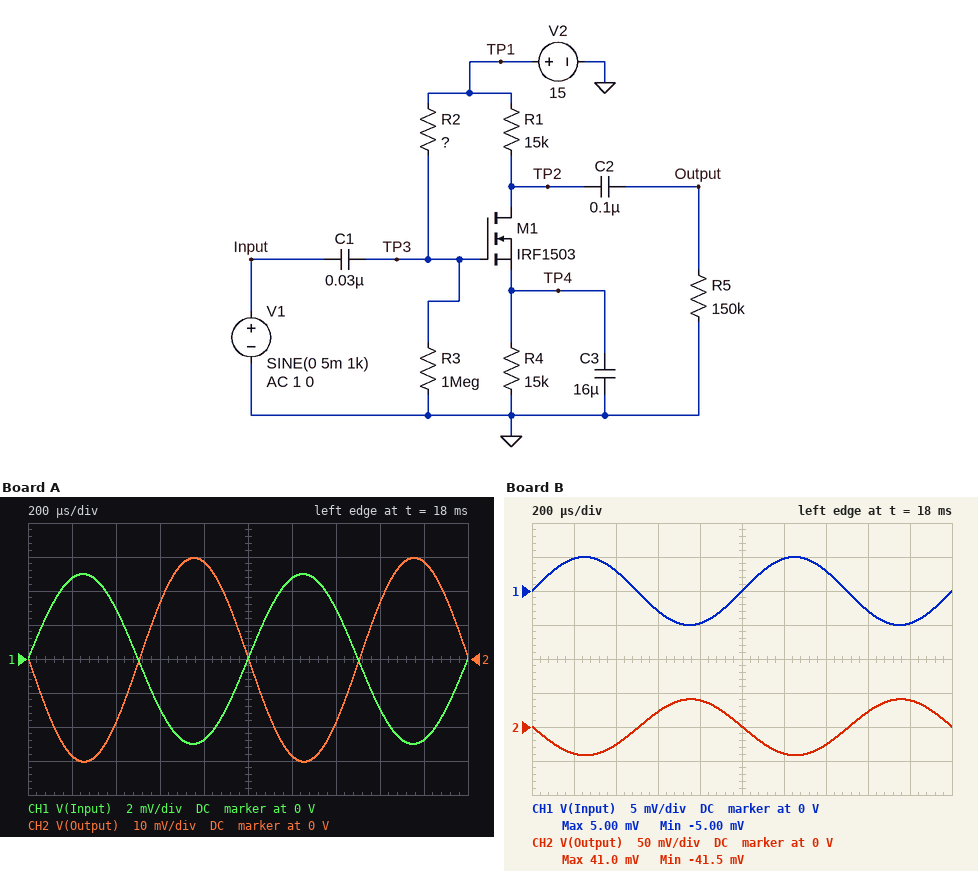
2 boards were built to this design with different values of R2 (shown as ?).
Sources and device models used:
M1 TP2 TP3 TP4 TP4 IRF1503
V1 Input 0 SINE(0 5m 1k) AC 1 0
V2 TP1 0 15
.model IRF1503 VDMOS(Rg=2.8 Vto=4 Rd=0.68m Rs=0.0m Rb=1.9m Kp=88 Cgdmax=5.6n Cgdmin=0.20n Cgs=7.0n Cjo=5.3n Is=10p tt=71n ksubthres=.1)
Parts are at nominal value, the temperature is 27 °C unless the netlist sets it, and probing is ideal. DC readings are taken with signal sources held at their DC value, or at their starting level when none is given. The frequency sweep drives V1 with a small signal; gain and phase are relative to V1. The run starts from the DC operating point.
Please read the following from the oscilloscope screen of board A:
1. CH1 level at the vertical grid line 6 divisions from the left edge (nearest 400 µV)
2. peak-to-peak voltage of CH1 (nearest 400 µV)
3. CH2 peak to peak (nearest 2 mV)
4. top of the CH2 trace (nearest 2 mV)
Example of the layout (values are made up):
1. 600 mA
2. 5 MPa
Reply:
1. 4.8 mV
2. 10.0 mV
3. 60 mV
4. 30 mV
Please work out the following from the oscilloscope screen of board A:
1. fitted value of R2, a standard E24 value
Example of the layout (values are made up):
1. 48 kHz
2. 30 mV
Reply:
1. 560 kΩ
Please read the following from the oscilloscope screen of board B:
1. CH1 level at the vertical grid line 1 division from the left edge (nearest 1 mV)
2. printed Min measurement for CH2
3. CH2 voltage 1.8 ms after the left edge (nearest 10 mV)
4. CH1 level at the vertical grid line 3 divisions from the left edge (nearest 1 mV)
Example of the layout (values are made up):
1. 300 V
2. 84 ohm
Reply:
1. 5 mV
2. -41.5 mV
3. 40 mV
4. -3 mV
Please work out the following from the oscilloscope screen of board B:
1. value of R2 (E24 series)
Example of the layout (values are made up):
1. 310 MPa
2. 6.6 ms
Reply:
1. 620 kΩ
